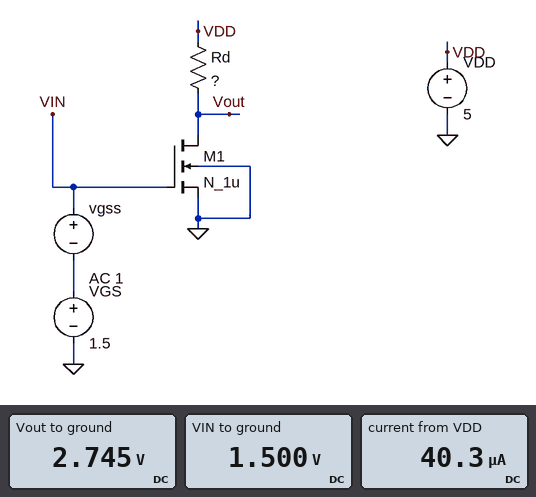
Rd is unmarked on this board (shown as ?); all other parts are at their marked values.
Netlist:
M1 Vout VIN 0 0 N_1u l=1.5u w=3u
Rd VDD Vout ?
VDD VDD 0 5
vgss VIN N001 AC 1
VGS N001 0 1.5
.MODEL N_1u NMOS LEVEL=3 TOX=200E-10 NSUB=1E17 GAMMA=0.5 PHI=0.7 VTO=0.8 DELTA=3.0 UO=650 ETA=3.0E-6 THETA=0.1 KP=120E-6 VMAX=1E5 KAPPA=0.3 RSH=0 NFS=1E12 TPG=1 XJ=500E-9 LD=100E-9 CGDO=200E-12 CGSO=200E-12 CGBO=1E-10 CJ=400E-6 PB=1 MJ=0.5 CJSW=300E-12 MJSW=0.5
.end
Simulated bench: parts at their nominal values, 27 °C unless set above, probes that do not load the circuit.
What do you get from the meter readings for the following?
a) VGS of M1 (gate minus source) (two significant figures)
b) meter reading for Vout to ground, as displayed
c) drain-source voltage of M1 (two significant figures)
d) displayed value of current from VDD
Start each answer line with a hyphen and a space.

- 1.5 V
- 2.745 V
- 2.7 V
- 40.3 µA
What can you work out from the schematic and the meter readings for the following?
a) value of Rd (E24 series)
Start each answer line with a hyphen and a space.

- 56 kΩ
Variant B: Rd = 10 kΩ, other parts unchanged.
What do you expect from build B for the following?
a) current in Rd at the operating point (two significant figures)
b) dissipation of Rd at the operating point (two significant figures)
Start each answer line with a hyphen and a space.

- 41 µA
- 17 µW
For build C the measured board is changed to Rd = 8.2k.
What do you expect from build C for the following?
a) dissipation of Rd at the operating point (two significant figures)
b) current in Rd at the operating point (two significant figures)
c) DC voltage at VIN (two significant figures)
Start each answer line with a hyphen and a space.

- 14 µW
- 41 µA
- 1.5 V
